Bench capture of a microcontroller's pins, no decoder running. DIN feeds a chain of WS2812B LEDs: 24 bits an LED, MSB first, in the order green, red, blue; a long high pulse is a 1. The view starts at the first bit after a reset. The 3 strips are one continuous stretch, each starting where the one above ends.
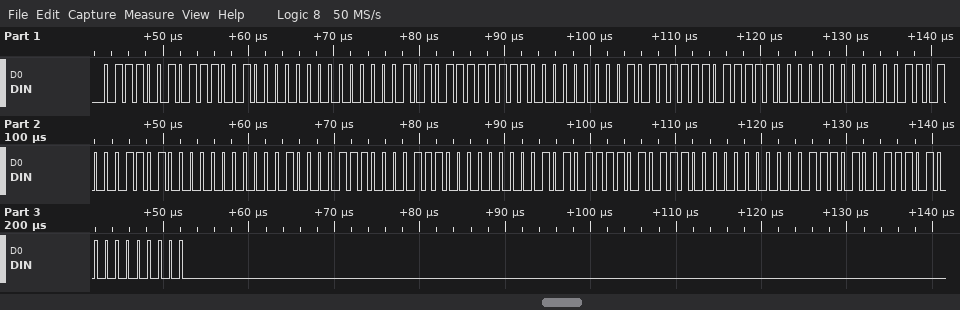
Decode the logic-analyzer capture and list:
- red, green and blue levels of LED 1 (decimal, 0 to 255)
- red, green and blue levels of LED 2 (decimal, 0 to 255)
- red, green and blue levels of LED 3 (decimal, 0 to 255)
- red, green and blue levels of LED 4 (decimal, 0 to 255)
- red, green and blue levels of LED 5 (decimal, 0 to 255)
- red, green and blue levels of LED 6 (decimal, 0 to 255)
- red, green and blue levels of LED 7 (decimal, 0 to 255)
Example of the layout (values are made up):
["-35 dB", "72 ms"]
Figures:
["228, 114, 0", "255, 10, 0", "190, 95, 0", "52, 26, 0", "135, 67, 0", "174, 87, 0", "116, 58, 0"]
